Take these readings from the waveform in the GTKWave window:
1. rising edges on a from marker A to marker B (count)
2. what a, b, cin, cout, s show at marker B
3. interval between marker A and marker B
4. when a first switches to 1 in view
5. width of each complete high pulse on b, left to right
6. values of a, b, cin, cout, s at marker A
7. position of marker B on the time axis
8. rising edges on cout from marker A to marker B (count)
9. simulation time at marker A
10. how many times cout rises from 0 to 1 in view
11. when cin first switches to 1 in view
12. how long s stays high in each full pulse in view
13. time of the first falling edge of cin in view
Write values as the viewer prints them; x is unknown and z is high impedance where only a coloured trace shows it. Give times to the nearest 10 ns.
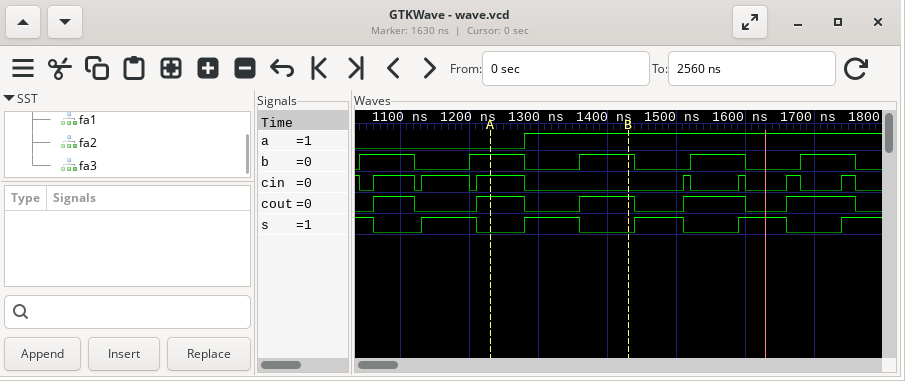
1
a=1, b=1, cin=0, cout=1, s=0
200 ns
1280 ns
80 ns, 80 ns, 80 ns, 80 ns, 80 ns
a=0, b=1, cin=1, cout=1, s=0
1430 ns
1
1230 ns
5
1060 ns
80 ns, 80 ns, 70 ns, 70 ns
1040 ns
